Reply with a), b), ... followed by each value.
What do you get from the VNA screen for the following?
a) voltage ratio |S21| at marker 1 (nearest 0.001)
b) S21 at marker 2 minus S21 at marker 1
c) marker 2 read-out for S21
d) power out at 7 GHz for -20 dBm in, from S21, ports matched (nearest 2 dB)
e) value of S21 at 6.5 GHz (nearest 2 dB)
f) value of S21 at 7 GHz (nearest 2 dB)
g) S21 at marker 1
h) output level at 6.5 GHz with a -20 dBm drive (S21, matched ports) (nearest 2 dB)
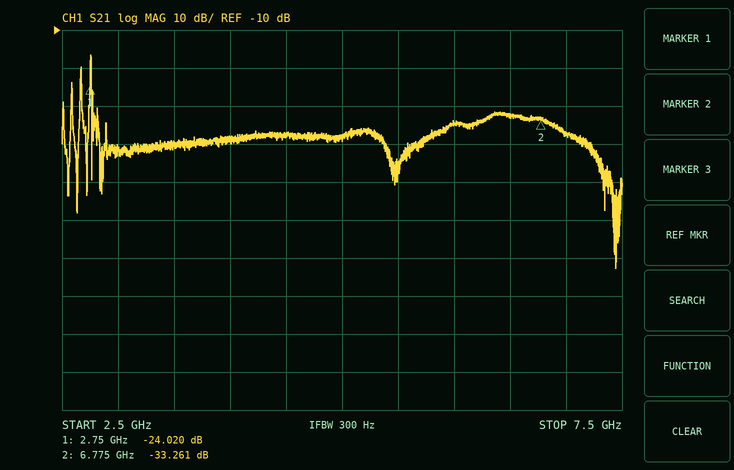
a) 0.063
b) -9.241 dB
c) -33.261 dB
d) -58 dBm
e) -32 dB
f) -38 dB
g) -24.020 dB
h) -52 dBm
